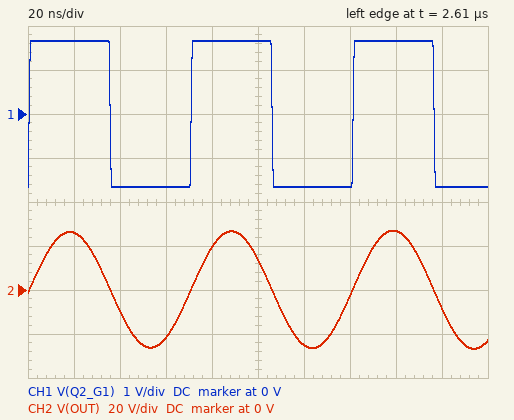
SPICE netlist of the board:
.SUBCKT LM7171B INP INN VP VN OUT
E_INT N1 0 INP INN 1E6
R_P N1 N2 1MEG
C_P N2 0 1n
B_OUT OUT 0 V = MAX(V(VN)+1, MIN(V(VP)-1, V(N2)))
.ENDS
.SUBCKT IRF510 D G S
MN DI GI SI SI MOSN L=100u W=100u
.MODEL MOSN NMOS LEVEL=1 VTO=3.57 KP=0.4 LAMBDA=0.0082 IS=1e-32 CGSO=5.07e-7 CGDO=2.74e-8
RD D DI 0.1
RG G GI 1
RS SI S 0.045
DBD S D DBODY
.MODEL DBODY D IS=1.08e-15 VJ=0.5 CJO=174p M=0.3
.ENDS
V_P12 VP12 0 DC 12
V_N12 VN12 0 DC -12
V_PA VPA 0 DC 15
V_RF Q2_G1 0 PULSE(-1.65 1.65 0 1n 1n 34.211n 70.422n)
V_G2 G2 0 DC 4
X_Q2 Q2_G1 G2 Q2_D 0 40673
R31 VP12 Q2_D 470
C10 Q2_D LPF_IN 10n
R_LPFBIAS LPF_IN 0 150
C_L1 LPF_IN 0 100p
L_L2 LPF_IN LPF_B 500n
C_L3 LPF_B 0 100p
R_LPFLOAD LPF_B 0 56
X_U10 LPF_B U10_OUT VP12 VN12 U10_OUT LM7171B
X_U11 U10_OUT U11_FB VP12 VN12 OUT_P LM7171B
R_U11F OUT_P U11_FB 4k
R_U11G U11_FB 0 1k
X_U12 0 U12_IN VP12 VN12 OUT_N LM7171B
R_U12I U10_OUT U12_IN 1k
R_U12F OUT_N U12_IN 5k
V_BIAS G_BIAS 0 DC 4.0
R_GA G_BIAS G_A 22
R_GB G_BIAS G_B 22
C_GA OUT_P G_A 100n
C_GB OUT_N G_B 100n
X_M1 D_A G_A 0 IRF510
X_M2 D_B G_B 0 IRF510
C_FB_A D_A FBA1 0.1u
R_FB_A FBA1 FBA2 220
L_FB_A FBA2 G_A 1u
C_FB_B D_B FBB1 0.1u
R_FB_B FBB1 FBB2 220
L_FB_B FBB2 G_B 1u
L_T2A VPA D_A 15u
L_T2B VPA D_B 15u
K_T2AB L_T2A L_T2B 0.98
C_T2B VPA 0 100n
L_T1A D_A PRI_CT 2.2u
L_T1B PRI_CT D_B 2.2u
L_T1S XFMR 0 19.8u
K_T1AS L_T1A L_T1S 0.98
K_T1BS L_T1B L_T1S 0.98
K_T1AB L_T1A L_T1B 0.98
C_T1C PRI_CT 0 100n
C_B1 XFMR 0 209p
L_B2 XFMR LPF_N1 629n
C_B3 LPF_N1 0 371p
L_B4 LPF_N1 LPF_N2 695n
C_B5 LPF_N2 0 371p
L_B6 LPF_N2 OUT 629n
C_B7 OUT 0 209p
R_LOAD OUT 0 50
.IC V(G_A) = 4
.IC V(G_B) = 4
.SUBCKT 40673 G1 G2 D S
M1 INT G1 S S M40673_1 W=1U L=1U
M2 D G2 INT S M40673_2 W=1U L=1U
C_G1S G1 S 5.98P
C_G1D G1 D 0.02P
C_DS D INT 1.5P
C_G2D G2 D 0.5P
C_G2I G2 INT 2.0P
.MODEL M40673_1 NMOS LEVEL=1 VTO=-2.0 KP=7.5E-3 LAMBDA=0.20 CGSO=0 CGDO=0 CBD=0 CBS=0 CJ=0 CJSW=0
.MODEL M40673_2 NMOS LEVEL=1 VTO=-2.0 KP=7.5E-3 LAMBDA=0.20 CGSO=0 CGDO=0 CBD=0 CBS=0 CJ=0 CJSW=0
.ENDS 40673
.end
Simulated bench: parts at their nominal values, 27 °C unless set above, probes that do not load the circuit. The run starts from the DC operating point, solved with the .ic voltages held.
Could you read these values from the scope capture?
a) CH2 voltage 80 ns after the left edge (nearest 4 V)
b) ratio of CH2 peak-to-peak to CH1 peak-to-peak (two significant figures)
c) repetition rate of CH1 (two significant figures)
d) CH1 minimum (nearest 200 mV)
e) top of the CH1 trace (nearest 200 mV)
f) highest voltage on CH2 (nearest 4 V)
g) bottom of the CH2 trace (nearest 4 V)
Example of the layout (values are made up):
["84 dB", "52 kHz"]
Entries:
["20 V", "16", "14 MHz", "-1.6 V", "1.6 V", "28 V", "-28 V"]
